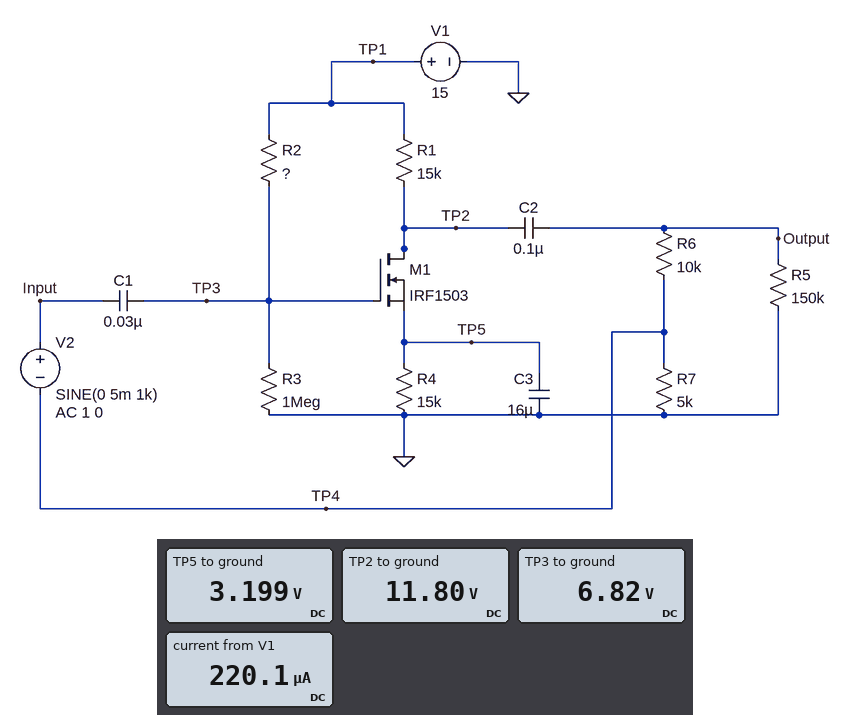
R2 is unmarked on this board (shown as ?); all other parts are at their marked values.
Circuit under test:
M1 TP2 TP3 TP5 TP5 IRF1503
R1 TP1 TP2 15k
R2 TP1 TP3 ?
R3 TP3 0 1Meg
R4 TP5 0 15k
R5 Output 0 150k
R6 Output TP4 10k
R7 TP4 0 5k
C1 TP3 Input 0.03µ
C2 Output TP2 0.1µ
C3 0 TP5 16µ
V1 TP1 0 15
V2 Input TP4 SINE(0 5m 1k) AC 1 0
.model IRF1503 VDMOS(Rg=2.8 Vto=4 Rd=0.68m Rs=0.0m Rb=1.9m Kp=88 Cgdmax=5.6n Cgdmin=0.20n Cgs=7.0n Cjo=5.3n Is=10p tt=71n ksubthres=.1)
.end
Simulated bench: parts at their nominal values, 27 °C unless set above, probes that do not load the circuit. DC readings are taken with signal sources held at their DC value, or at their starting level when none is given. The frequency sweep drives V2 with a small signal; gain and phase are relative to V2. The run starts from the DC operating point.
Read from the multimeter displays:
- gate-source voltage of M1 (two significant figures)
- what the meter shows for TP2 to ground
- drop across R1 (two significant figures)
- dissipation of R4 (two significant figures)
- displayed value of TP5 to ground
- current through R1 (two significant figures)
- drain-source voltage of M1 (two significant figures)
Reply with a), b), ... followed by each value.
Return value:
a) 3.6 V
b) 11.80 V
c) 3.2 V
d) 680 µW
e) 3.199 V
f) 210 µA
g) 8.6 V
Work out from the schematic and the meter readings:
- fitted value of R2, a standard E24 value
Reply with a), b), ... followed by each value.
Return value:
a) 1.2 MΩ
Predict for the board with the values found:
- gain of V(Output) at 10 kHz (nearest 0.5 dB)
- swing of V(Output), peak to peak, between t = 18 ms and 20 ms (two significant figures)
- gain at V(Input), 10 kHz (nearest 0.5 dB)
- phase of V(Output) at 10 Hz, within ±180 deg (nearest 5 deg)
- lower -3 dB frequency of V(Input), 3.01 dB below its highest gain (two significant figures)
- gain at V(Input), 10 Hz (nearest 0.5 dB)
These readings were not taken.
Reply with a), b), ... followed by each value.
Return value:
a) 7.5 dB
b) 25 mV
c) -15.0 dB
d) 5 deg
e) 9.8 Hz
f) 3.0 dB
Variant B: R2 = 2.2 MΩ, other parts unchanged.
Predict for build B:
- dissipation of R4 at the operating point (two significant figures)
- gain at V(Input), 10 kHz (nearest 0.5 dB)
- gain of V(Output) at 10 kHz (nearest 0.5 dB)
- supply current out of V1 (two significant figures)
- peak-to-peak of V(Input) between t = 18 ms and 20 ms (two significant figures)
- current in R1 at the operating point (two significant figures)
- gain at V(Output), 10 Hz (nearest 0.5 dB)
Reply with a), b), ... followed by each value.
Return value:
a) 84 µW
b) -10.0 dB
c) 6.0 dB
d) 79 µA
e) 2.8 mV
f) 75 µA
g) 0 dB
